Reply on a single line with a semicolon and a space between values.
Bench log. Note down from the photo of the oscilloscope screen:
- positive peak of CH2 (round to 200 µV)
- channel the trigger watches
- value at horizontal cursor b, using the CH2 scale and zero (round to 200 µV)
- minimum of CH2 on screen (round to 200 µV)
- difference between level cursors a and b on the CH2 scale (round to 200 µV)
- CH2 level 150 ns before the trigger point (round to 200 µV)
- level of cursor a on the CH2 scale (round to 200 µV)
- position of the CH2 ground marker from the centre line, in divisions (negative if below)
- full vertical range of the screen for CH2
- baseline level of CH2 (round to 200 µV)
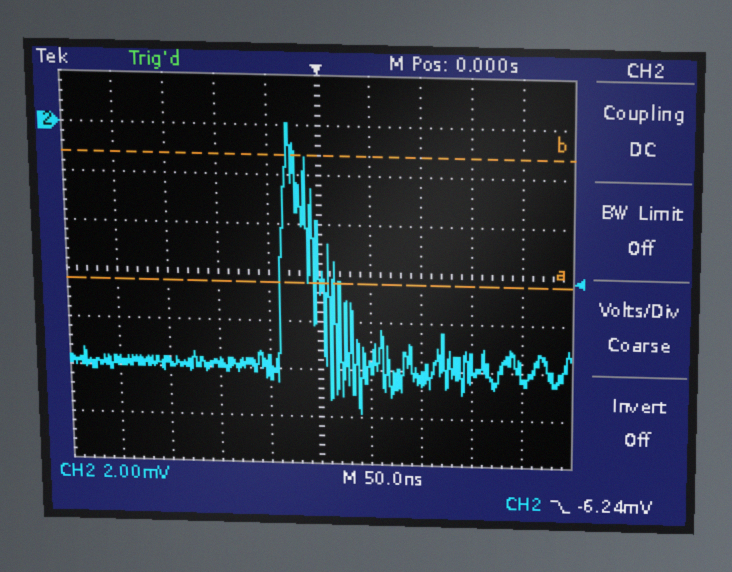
0.0 mV; CH2; -1.2 mV; -11.8 mV; 5.2 mV; -9.8 mV; -6.4 mV; +3.0 div; 16 mV; -9.8 mV
